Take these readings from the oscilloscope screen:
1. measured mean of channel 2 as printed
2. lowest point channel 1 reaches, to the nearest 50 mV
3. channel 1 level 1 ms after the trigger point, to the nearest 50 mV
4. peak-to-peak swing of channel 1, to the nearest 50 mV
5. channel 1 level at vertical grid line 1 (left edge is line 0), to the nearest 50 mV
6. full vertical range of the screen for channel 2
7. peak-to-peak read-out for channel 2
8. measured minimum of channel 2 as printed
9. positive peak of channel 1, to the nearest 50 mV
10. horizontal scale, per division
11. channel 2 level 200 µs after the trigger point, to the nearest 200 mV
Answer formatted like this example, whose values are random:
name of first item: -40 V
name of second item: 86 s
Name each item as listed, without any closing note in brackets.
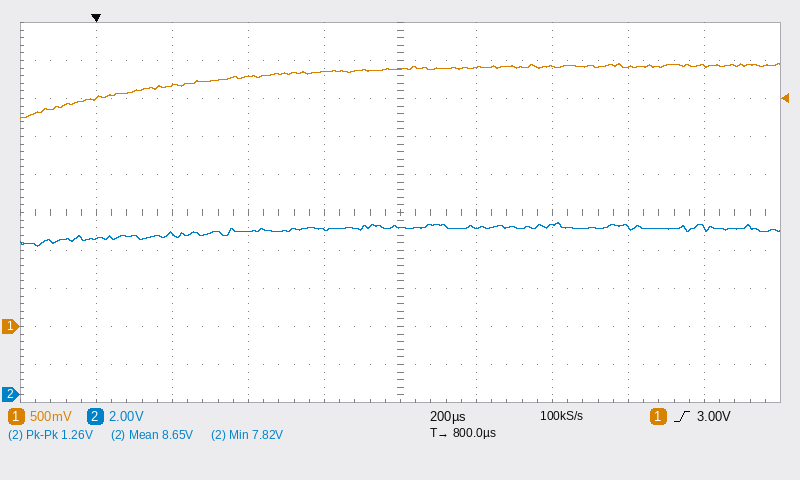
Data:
measured mean of channel 2 as printed: 8.65 V
lowest point channel 1 reaches, to the nearest 50 mV: 2.75 V
channel 1 level 1 ms after the trigger point, to the nearest 50 mV: 3.40 V
peak-to-peak swing of channel 1, to the nearest 50 mV: 700 mV
channel 1 level at vertical grid line 1 (left edge is line 0), to the nearest 50 mV: 3.00 V
full vertical range of the screen for channel 2: 20 V
peak-to-peak read-out for channel 2: 1.26 V
measured minimum of channel 2 as printed: 7.82 V
positive peak of channel 1, to the nearest 50 mV: 3.45 V
horizontal scale, per division: 200 µs
channel 2 level 200 µs after the trigger point, to the nearest 200 mV: 8.4 V
